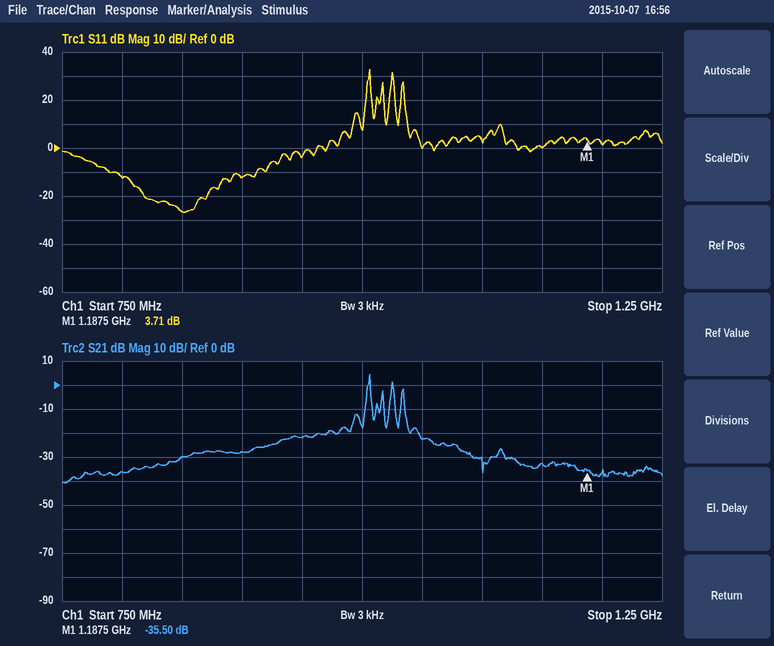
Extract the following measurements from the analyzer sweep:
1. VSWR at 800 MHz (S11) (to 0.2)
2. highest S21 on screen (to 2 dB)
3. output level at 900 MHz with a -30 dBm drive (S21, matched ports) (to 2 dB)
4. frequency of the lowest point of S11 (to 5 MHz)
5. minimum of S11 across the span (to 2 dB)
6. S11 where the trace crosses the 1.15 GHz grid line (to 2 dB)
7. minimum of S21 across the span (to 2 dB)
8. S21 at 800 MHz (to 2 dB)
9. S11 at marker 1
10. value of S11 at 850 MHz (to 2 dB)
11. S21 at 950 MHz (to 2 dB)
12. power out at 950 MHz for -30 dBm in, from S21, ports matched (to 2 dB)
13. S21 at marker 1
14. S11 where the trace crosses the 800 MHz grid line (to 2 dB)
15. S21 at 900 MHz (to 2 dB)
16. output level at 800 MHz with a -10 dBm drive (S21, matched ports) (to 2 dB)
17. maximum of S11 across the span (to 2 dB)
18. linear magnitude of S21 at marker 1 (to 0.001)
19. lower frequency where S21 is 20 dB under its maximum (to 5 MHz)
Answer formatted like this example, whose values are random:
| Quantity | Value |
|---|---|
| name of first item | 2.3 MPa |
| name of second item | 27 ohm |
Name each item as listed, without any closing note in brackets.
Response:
| Quantity | Value |
|---|---|
| VSWR at 800 MHz (S11) | 1.6 |
| highest S21 on screen | 4 dB |
| output level at 900 MHz with a -30 dBm drive (S21, matched ports) | -58 dBm |
| frequency of the lowest point of S11 | 850 MHz |
| minimum of S11 across the span | -26 dB |
| S11 where the trace crosses the 1.15 GHz grid line | 0 dB |
| minimum of S21 across the span | -40 dB |
| S21 at 800 MHz | -36 dB |
| S11 at marker 1 | 3.71 dB |
| value of S11 at 850 MHz | -26 dB |
| S21 at 950 MHz | -22 dB |
| power out at 950 MHz for -30 dBm in, from S21, ports matched | -52 dBm |
| S21 at marker 1 | -35.50 dB |
| S11 where the trace crosses the 800 MHz grid line | -12 dB |
| S21 at 900 MHz | -28 dB |
| output level at 800 MHz with a -10 dBm drive (S21, matched ports) | -46 dBm |
| maximum of S11 across the span | 32 dB |
| linear magnitude of S21 at marker 1 | 0.017 |
| lower frequency where S21 is 20 dB under its maximum | 1.000 GHz |
